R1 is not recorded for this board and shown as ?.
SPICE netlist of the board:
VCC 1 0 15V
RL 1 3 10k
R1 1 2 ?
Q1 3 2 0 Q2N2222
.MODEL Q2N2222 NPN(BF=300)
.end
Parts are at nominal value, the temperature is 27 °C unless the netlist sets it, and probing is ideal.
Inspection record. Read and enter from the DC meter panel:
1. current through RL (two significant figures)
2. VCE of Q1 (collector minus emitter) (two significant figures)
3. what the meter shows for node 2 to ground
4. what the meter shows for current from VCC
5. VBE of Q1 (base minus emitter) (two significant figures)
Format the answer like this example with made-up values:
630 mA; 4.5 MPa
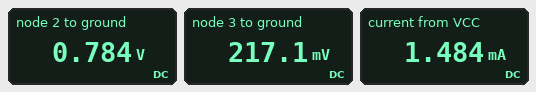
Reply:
1.5 mA; 220 mV; 0.784 V; 1.484 mA; 780 mV
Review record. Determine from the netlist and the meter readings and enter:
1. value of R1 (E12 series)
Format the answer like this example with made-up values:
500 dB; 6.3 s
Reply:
2.7 MΩ
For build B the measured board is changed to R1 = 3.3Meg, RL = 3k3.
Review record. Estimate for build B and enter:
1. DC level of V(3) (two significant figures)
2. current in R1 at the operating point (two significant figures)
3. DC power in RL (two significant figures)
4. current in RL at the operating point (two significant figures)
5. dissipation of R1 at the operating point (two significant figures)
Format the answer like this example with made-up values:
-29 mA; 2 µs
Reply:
11 V; 4.3 µA; 5.5 mW; 1.3 mA; 61 µW
